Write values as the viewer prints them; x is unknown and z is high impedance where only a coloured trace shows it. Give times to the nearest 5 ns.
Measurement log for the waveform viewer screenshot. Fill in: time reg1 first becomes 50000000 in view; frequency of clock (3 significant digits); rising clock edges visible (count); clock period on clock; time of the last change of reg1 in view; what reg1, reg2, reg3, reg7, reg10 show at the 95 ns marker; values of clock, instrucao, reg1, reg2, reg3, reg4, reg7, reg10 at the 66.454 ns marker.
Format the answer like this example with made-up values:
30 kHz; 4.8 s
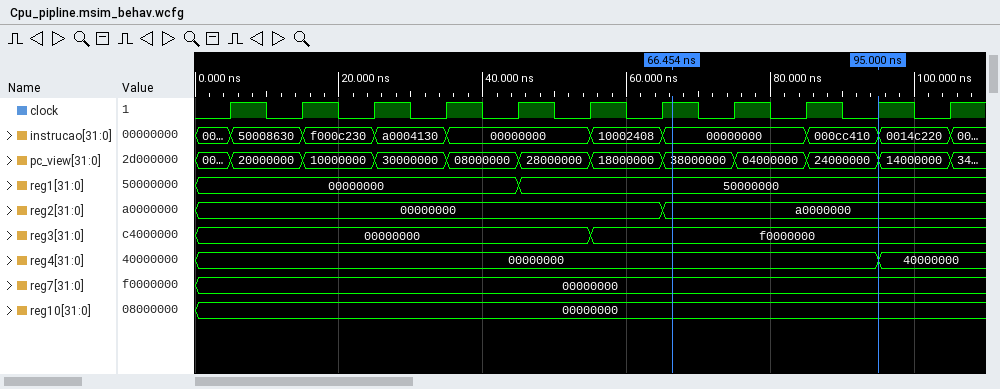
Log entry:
45 ns; 100 MHz; 11; 10 ns; 45 ns; reg1=50000000, reg2=a0000000, reg3=f0000000, reg7=00000000, reg10=00000000; clock=1, instrucao=00000000, reg1=50000000, reg2=a0000000, reg3=f0000000, reg4=00000000, reg7=00000000, reg10=00000000
